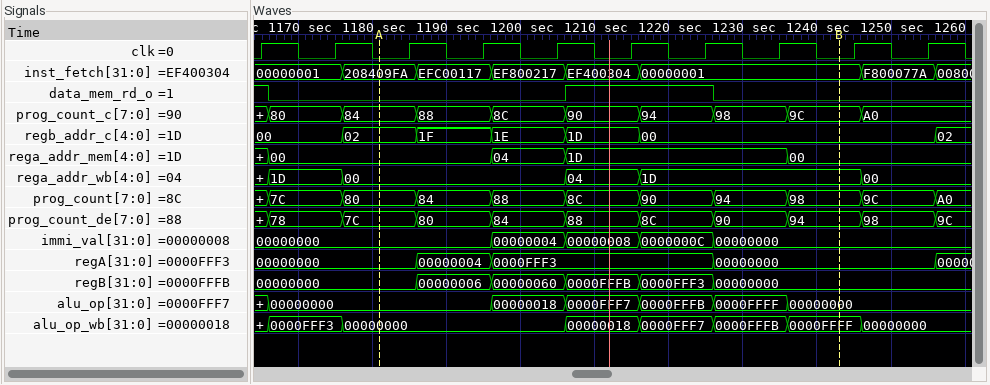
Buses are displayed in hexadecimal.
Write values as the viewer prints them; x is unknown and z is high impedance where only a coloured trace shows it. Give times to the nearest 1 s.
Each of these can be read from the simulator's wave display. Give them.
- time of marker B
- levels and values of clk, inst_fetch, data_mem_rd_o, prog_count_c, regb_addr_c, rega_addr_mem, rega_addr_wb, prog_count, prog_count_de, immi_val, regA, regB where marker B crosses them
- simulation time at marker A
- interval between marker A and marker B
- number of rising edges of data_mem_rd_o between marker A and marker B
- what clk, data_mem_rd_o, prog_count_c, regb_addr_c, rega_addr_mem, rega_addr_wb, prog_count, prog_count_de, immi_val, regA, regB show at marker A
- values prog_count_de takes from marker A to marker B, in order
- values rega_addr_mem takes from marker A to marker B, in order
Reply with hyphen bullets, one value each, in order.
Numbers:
- 1243 s
- clk=0, inst_fetch=00000001, data_mem_rd_o=0, prog_count_c=9C, regb_addr_c=00, rega_addr_mem=00, rega_addr_wb=1D, prog_count=98, prog_count_de=94, immi_val=00000000, regA=00000000, regB=00000000
- 1181 s
- 62 s
- 1
- clk=0, data_mem_rd_o=0, prog_count_c=84, regb_addr_c=02, rega_addr_mem=00, rega_addr_wb=00, prog_count=80, prog_count_de=7C, immi_val=00000000, regA=00000000, regB=00000000
- 7C, 80, 84, 88, 8C, 90, 94
- 00, 04, 1D, 00
